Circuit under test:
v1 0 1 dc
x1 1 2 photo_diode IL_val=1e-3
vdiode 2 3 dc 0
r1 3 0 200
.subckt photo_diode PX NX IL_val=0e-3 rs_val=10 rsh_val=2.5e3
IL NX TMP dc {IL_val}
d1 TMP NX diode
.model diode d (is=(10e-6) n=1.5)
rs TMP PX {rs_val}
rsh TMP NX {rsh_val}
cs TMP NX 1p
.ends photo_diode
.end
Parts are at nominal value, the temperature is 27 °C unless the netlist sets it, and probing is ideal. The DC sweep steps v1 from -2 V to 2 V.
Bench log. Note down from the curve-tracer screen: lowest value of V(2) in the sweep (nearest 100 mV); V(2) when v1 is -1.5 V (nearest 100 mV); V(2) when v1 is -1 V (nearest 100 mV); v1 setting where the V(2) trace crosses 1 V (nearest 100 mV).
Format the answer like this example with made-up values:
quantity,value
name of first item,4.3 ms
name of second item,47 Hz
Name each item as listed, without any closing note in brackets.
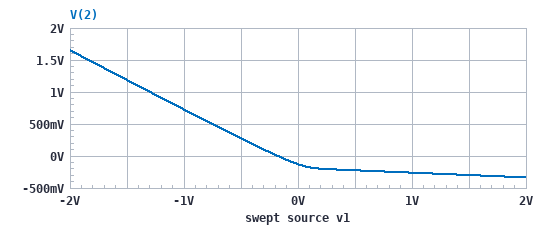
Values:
quantity,value
lowest value of V(2) in the sweep,-300 mV
V(2) when v1 is -1.5 V,1.2 V
V(2) when v1 is -1 V,700 mV
v1 setting where the V(2) trace crosses 1 V,-1.3 V
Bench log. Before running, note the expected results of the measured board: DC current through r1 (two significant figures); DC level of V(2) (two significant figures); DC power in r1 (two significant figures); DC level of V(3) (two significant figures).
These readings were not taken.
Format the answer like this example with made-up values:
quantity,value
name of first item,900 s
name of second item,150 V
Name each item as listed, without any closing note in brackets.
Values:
quantity,value
DC current through r1,640 µA
DC level of V(2),-130 mV
DC power in r1,82 µW
DC level of V(3),-130 mV
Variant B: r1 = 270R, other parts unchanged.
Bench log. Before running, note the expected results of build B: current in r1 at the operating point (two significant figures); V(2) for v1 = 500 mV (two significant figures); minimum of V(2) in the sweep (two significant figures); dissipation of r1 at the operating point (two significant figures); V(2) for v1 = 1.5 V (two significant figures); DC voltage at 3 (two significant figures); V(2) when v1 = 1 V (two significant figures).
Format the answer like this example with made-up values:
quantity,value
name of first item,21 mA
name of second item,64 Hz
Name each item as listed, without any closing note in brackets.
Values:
quantity,value
current in r1 at the operating point,520 µA
V(2) for v1 = 500 mV,-290 mV
minimum of V(2) in the sweep,-440 mV
dissipation of r1 at the operating point,73 µW
V(2) for v1 = 1.5 V,-390 mV
DC voltage at 3,-140 mV
V(2) when v1 = 1 V,-340 mV
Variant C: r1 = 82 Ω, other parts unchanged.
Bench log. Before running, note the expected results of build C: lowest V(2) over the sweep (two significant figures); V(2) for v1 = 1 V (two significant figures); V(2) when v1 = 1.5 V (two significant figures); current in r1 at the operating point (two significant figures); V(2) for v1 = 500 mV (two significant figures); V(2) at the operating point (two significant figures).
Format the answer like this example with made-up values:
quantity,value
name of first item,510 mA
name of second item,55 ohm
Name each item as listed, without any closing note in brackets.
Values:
quantity,value
lowest V(2) over the sweep,-140 mV
V(2) for v1 = 1 V,-110 mV
V(2) when v1 = 1.5 V,-130 mV
current in r1 at the operating point,890 µA
V(2) for v1 = 500 mV,-96 mV
V(2) at the operating point,-73 mV
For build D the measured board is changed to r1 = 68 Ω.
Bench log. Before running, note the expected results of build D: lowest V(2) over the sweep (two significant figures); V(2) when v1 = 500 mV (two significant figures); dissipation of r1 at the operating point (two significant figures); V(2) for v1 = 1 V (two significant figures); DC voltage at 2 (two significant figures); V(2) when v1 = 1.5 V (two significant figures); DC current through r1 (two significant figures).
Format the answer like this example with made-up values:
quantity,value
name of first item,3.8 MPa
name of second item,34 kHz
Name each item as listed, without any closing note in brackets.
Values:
quantity,value
lowest V(2) over the sweep,-120 mV
V(2) when v1 = 500 mV,-80 mV
dissipation of r1 at the operating point,57 µW
V(2) for v1 = 1 V,-93 mV
DC voltage at 2,-62 mV
V(2) when v1 = 1.5 V,-110 mV
DC current through r1,920 µA
